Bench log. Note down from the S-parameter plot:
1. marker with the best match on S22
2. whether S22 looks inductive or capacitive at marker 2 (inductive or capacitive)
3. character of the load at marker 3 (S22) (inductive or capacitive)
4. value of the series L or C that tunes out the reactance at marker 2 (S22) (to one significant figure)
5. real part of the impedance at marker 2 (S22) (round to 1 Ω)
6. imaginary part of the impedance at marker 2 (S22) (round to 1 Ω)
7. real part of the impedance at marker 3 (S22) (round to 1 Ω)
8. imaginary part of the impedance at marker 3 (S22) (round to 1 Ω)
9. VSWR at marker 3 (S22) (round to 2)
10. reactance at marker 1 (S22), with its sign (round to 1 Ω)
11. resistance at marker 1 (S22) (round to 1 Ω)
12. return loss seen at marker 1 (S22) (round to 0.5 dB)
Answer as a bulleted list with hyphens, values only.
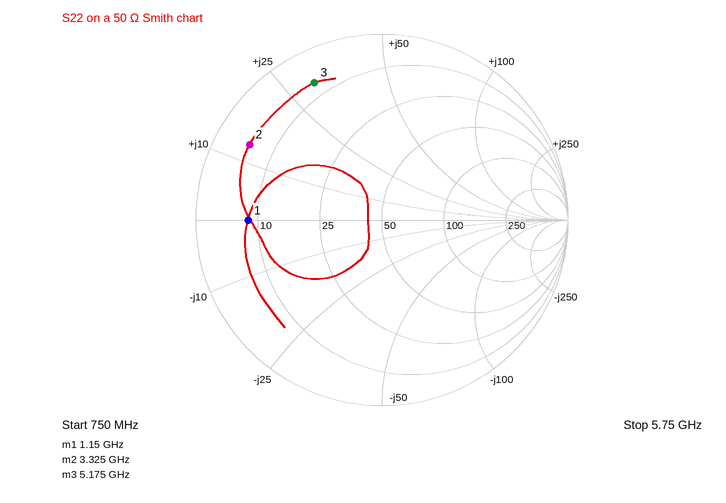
- marker 1
- inductive
- inductive
- 4 pF
- 5 Ω
- +13 Ω
- 7 Ω
- +31 Ω
- 10
- 0 Ω
- 8 Ω
- 3.0 dB
